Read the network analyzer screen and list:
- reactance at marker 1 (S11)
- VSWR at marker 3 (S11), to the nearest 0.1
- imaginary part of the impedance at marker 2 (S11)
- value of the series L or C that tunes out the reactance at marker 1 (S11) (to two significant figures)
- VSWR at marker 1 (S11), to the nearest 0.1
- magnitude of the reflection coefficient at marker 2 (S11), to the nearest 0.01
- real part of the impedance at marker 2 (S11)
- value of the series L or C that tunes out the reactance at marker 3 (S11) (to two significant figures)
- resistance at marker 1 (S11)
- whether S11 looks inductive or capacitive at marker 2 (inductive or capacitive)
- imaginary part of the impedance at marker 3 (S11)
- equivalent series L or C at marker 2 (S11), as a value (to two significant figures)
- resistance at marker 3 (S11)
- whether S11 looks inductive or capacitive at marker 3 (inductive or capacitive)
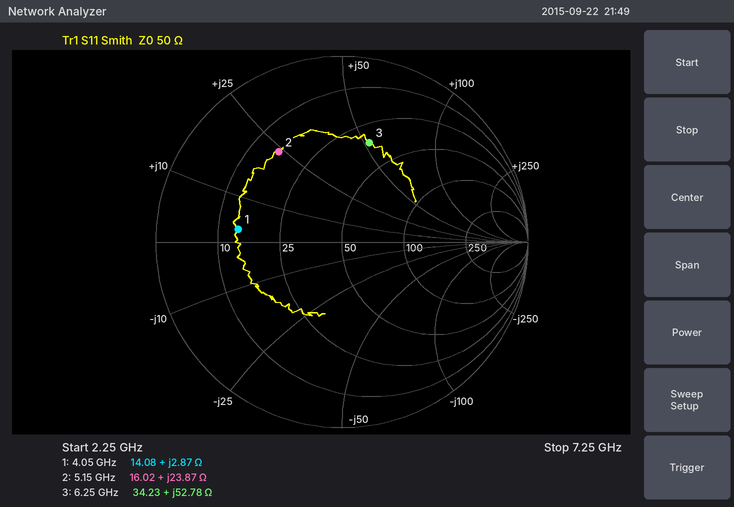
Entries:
+2.87 Ω
3.5
+23.87 Ω
14 pF
3.6
0.59
16.02 Ω
480 fF
14.08 Ω
inductive
+52.78 Ω
740 pH
34.23 Ω
inductive
